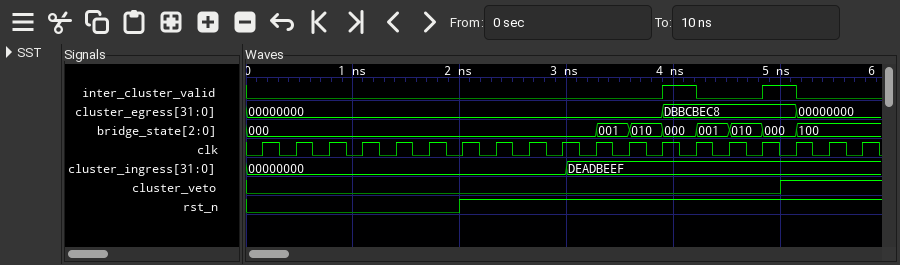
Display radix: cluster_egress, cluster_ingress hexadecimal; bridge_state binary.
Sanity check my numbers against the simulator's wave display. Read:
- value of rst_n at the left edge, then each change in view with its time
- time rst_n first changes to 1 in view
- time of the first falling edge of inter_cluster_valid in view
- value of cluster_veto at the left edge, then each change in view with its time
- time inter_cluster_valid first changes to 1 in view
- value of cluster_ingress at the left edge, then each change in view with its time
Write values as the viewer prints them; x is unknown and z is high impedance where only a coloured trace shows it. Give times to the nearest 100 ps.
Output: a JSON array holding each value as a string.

["0, 1 at 2000 ps", "2000 ps", "4200 ps", "0, 1 at 5000 ps", "3900 ps", "00000000, DEADBEEF at 3000 ps"]
